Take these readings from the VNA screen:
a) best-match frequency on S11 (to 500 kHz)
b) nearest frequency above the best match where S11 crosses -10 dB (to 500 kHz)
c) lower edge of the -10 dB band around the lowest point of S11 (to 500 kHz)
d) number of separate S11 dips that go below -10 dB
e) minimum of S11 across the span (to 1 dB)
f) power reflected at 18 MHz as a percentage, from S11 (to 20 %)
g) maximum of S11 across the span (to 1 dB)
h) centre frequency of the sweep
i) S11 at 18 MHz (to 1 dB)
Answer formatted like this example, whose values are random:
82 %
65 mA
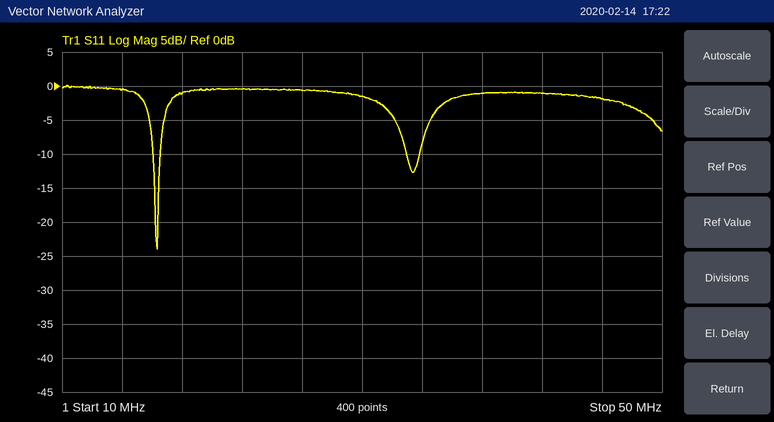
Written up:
16.5 MHz
16.5 MHz
16.0 MHz
2
-24 dB
80 %
0 dB
30 MHz
-1 dB
